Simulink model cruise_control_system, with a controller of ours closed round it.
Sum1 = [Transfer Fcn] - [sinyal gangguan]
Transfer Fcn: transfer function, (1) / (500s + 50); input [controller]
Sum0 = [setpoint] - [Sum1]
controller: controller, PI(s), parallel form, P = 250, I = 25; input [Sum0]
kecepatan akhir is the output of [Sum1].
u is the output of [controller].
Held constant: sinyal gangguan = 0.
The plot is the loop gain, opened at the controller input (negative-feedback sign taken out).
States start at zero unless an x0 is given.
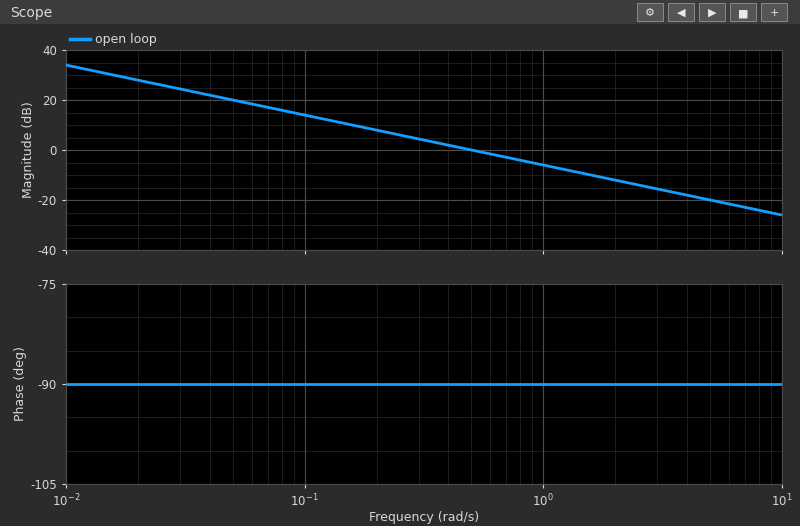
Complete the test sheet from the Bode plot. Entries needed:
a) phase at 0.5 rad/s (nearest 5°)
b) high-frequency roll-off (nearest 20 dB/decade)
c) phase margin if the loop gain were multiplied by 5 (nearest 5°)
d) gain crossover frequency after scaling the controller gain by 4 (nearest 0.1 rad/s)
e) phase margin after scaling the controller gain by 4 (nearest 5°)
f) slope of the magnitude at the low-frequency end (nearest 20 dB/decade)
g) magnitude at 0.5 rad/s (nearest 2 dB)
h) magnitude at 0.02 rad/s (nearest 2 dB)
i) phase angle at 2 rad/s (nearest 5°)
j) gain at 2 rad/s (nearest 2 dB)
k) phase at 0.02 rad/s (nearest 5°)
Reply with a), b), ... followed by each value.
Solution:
a) -90°
b) -20 dB/decade
c) 90°
d) 2.0 rad/s
e) 90°
f) -20 dB/decade
g) 0 dB
h) 28 dB
i) -90°
j) -12 dB
k) -90°
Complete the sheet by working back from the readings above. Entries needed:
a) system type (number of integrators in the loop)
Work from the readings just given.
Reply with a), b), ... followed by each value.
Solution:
a) 1
